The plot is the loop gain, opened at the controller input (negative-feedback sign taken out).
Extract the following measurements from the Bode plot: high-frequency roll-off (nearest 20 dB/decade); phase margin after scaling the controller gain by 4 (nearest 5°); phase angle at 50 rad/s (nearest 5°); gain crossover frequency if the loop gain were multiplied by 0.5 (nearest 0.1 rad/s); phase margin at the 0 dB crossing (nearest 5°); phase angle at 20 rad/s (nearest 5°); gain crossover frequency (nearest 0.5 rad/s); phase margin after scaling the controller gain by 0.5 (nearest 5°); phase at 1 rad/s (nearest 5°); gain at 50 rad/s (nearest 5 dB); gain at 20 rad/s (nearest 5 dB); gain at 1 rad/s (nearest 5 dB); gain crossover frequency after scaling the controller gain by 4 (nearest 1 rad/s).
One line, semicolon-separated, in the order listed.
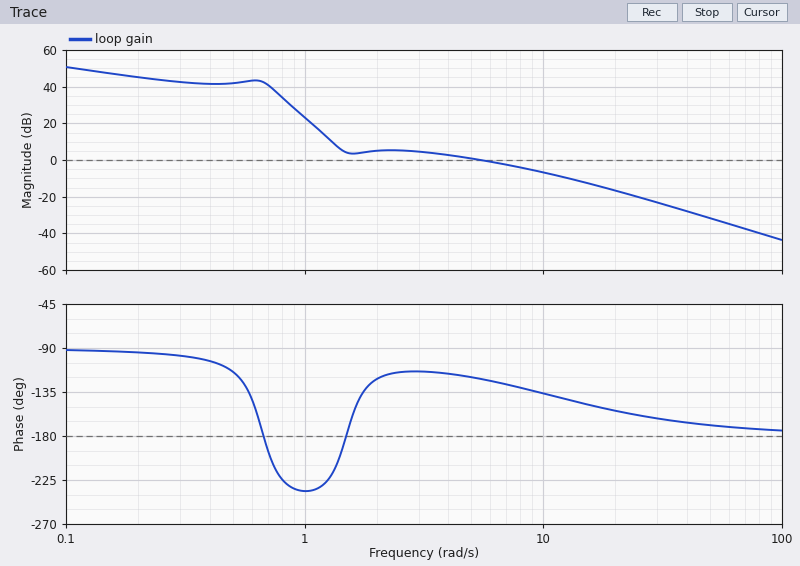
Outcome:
-40 dB/decade; 35°; -170°; 1.4 rad/s; 60°; -155°; 5.5 rad/s; -20°; -235°; -30 dB; -15 dB; 25 dB; 15 rad/s
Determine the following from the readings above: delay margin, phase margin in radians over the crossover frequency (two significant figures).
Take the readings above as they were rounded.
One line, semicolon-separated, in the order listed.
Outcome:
0.19 s
